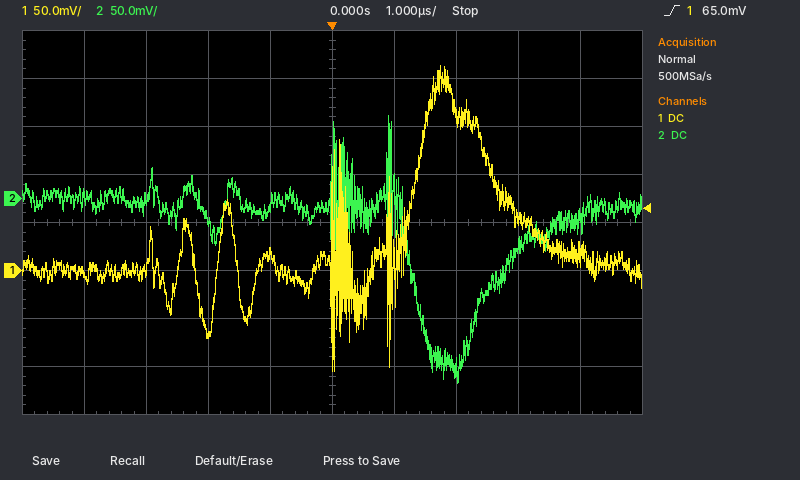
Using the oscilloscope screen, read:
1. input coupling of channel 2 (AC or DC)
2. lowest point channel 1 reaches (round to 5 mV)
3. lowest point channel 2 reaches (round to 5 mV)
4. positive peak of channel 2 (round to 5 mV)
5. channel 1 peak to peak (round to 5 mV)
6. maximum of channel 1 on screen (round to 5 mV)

DC
-105 mV
-190 mV
85 mV
320 mV
215 mV
